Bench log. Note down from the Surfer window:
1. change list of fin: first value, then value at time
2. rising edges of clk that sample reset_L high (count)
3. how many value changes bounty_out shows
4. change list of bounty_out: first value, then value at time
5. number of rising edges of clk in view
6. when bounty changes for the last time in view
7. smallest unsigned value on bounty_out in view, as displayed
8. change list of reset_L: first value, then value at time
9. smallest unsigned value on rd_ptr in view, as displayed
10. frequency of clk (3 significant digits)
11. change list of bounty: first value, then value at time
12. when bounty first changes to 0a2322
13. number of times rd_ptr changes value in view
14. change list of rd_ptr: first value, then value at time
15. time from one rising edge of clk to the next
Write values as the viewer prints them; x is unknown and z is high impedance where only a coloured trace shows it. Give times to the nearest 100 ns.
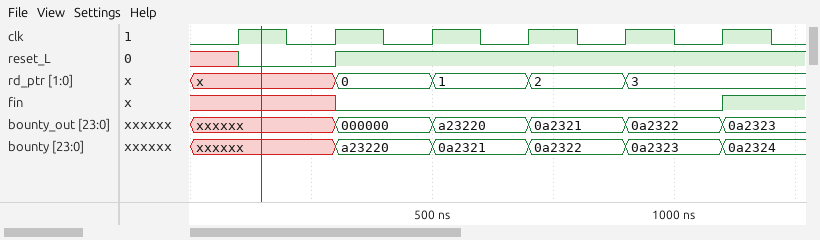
x, 0 at 300 ns, 1 at 1100 ns
4
5
xxxxxx, 000000 at 300 ns, a23220 at 500 ns, 0a2321 at 700 ns, 0a2322 at 900 ns, 0a2323 at 1100 ns
6
1100 ns
000000
x, 0 at 100 ns, 1 at 300 ns
0
5.00 MHz
xxxxxx, a23220 at 300 ns, 0a2321 at 500 ns, 0a2322 at 700 ns, 0a2323 at 900 ns, 0a2324 at 1100 ns
700 ns
4
x, 0 at 300 ns, 1 at 500 ns, 2 at 700 ns, 3 at 900 ns
200 ns
